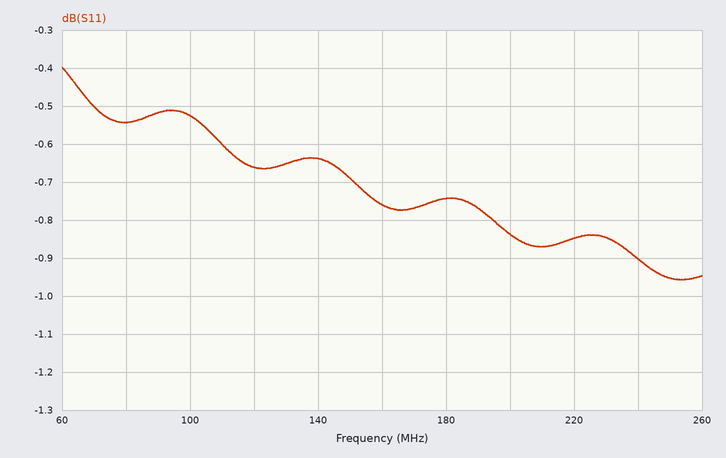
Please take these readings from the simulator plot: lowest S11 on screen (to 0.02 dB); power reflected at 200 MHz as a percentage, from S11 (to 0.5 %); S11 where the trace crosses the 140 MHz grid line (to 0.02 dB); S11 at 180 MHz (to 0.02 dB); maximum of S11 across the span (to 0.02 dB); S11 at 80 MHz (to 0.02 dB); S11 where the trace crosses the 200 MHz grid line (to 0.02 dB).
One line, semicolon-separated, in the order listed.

-0.96 dB; 82.5 %; -0.64 dB; -0.74 dB; -0.40 dB; -0.54 dB; -0.84 dB
